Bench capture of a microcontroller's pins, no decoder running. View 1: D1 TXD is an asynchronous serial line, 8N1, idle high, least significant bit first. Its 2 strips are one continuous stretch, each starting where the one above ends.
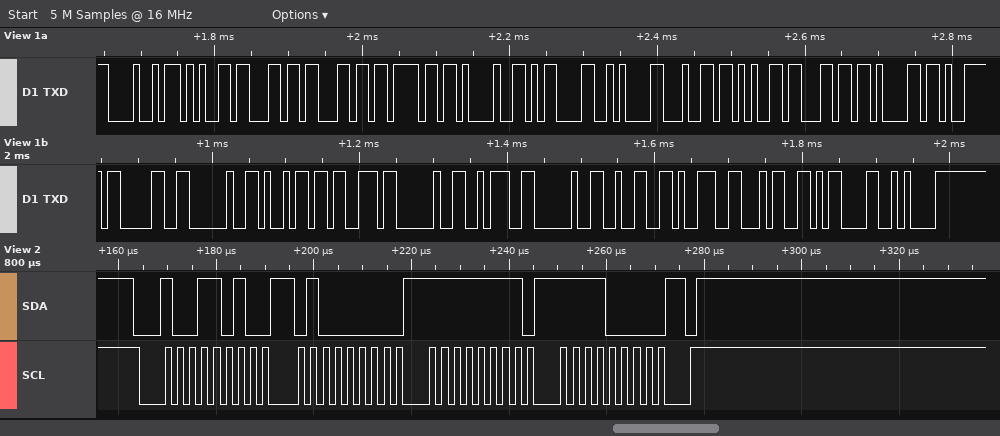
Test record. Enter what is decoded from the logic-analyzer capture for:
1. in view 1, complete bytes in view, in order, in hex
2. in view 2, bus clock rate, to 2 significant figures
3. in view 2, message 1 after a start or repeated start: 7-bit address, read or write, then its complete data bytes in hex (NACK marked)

48 65 6C 6C 6F 21 0D 0A 64 65 6C 61 79 30 20 69 73 20 3A 20 32 39 34 0D 0A
400 kHz
0x4D write: 40 FF F0
